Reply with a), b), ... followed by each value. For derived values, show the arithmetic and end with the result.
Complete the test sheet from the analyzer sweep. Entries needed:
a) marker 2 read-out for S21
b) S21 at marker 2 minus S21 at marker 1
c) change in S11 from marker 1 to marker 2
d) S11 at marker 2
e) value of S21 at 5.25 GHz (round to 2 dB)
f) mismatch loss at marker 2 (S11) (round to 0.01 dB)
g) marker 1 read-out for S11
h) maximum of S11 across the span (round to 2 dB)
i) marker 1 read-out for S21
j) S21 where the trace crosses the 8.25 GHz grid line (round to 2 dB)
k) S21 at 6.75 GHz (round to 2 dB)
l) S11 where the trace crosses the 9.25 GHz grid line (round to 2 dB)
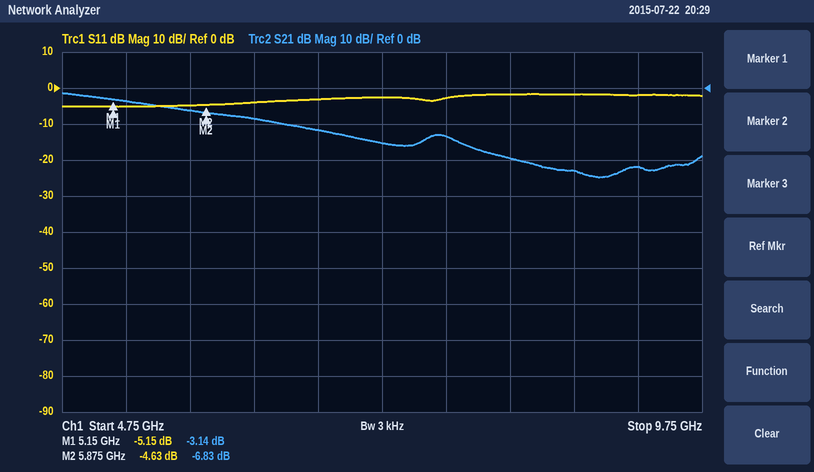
a) -6.83 dB
b) -6.83 − (-3.14) = -3.69 dB
c) -4.63 − (-5.15) = 0.52 dB
d) -4.63 dB
e) -4 dB
f) −10 log10(1 − 10^(-4.63/10)) ≈ 1.83 dB
g) -5.15 dB
h) -2 dB
i) -3.14 dB
j) -20 dB
k) -12 dB
l) -2 dB
